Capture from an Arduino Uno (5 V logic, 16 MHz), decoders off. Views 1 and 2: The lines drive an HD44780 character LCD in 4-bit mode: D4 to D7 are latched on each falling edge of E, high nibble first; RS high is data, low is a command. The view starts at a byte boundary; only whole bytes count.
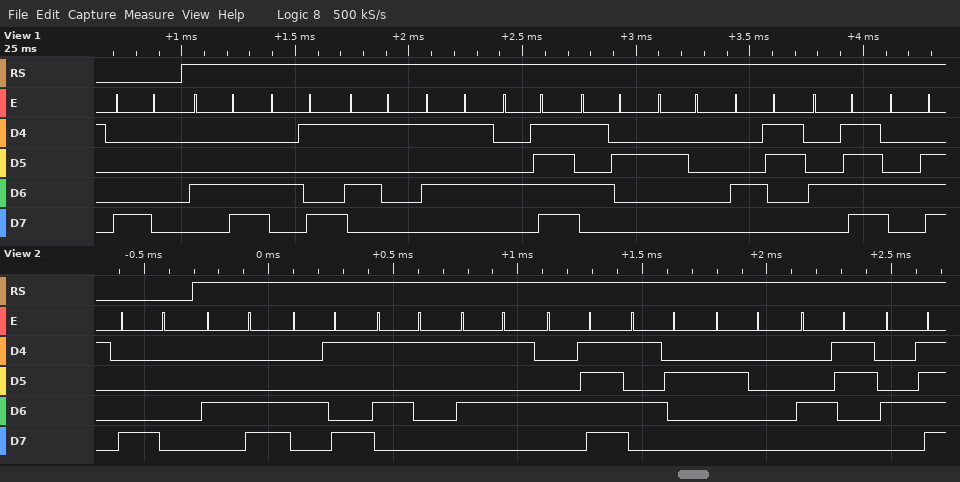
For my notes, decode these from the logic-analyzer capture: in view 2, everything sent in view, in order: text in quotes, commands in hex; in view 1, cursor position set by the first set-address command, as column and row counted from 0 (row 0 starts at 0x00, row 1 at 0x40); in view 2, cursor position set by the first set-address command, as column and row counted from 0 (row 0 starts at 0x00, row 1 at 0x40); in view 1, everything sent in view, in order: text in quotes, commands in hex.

0x80 "LIQUOR CO"
column 0, row 0
column 0, row 0
0x80 "LIQUOR CON"
